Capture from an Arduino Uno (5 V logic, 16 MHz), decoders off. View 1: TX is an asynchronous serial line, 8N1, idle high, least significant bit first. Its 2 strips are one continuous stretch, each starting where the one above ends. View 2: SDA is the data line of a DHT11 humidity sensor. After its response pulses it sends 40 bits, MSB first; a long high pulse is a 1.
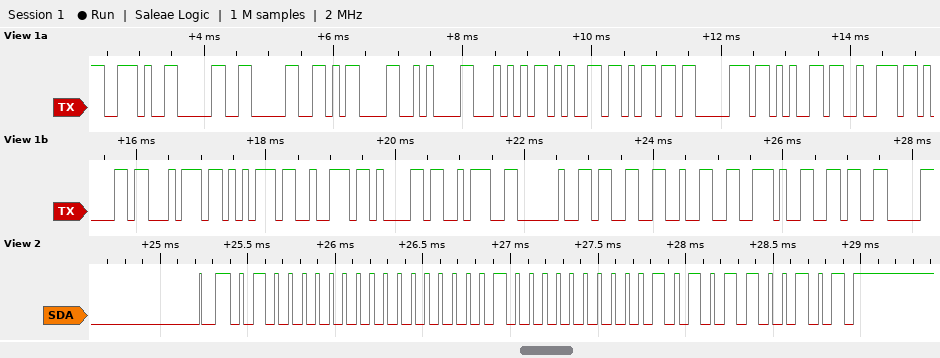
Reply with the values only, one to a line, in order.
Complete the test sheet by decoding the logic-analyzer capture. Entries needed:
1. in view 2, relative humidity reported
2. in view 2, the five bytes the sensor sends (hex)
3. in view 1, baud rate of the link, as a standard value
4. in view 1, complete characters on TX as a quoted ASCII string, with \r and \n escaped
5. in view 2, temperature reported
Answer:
64 %
40 00 20 05 65
9600 baud
".00\r\nTemperatura: 32.6"
32.5 °C
